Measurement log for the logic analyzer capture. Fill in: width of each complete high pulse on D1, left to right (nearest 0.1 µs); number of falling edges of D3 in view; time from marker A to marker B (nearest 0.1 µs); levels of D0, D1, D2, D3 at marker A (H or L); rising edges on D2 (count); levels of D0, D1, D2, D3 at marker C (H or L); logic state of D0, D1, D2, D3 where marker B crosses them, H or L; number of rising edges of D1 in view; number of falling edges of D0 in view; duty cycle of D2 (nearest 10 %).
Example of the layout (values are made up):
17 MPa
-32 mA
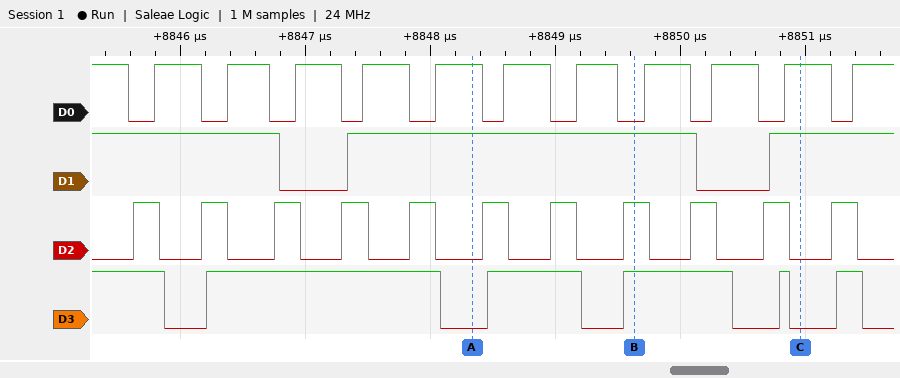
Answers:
2.8 µs
6
1.3 µs
D0=H, D1=H, D2=L, D3=L
11
D0=H, D1=H, D2=L, D3=L
D0=L, D1=H, D2=H, D3=H
2
11
40 %
